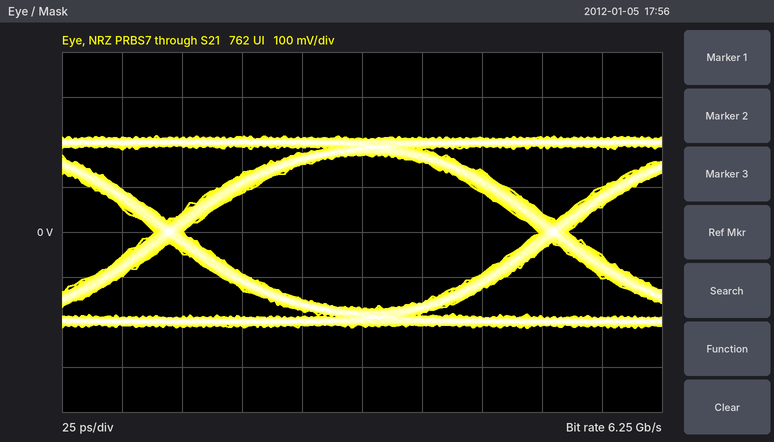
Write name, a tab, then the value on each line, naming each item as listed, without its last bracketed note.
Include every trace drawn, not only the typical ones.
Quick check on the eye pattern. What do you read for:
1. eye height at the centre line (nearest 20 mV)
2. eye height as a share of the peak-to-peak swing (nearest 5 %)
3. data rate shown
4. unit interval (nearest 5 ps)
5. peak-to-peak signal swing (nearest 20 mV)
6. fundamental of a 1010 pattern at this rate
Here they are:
eye height at the centre line	340 mV
eye height as a share of the peak-to-peak swing	80 %
data rate shown	6.25 Gb/s
unit interval	160 ps
peak-to-peak signal swing	420 mV
fundamental of a 1010 pattern at this rate	3.125 GHz
